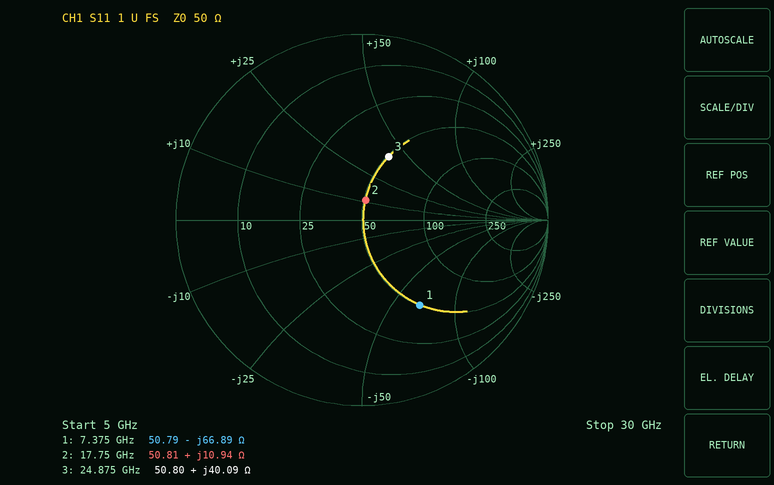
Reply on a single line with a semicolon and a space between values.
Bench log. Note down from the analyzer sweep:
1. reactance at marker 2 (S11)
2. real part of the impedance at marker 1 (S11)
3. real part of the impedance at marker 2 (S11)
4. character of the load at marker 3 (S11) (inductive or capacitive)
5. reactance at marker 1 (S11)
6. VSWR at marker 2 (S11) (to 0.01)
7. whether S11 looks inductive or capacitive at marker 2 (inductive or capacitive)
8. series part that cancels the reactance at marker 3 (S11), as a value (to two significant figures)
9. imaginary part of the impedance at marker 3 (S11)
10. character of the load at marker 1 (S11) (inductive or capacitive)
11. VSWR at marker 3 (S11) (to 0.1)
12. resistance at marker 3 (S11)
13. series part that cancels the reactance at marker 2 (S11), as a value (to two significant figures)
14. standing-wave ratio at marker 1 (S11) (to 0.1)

+10.94 Ω; 50.79 Ω; 50.81 Ω; inductive; -66.89 Ω; 1.24; inductive; 160 fF; +40.09 Ω; capacitive; 2.2; 50.80 Ω; 820 fF; 3.5
